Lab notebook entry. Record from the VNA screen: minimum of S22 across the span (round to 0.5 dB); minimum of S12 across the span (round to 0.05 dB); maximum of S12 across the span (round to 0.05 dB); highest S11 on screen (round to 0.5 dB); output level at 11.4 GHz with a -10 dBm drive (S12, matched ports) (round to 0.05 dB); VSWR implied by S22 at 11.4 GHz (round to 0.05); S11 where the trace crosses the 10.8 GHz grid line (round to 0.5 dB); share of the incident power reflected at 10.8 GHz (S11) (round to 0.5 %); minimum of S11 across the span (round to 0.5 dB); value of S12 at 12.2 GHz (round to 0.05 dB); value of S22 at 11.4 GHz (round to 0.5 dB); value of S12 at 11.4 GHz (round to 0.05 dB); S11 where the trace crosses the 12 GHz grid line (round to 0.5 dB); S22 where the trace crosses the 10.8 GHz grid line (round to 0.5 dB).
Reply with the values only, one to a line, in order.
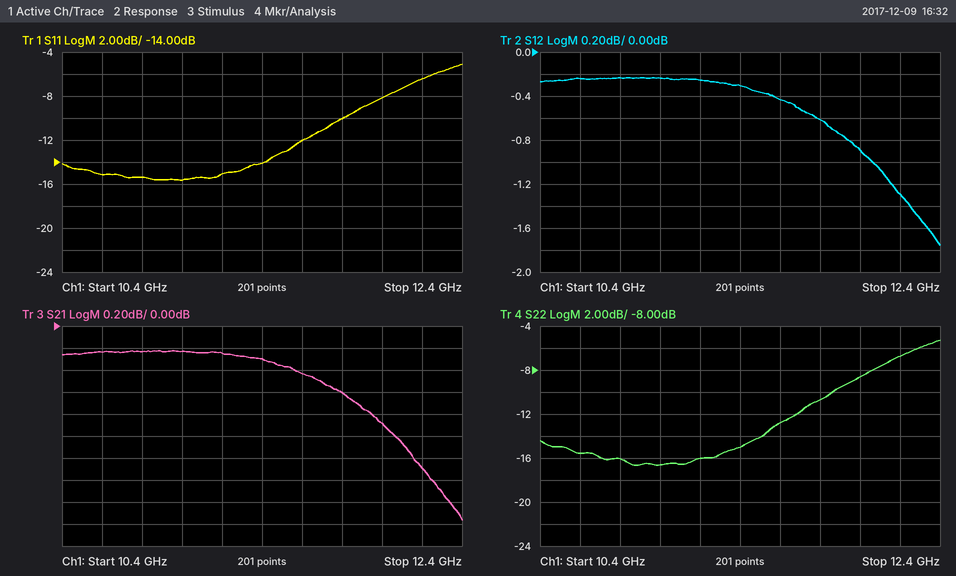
-16.5 dB
-1.75 dB
-0.25 dB
-5.0 dB
-10.30 dBm
1.45
-15.5 dB
3.0 %
-15.5 dB
-1.30 dB
-15.0 dB
-0.30 dB
-8.0 dB
-16.0 dB
